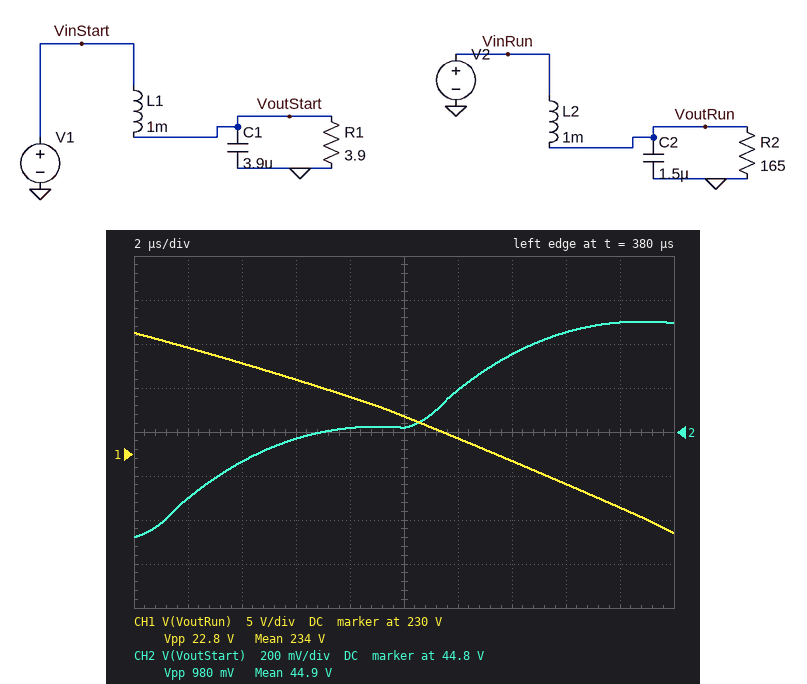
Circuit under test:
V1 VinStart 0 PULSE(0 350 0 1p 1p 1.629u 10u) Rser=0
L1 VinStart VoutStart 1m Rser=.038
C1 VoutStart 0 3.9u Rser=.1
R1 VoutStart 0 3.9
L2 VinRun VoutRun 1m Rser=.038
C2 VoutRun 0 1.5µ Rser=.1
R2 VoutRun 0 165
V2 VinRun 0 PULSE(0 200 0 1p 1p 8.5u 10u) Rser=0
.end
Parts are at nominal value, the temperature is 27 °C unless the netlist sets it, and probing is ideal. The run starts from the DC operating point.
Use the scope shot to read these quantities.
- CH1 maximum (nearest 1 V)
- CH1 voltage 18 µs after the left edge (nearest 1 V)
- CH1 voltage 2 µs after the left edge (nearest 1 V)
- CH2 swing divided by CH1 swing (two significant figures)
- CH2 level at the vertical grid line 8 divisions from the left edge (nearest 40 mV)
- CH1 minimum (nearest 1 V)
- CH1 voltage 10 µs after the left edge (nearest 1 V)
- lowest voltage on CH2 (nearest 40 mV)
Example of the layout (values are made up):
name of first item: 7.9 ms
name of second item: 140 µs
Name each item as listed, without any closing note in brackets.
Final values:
CH1 maximum: 244 V
CH1 voltage 18 µs after the left edge: 224 V
CH1 voltage 2 µs after the left edge: 242 V
CH2 swing divided by CH1 swing: 0.043
CH2 level at the vertical grid line 8 divisions from the left edge: 45.24 V
CH1 minimum: 221 V
CH1 voltage 10 µs after the left edge: 234 V
lowest voltage on CH2: 44.32 V
